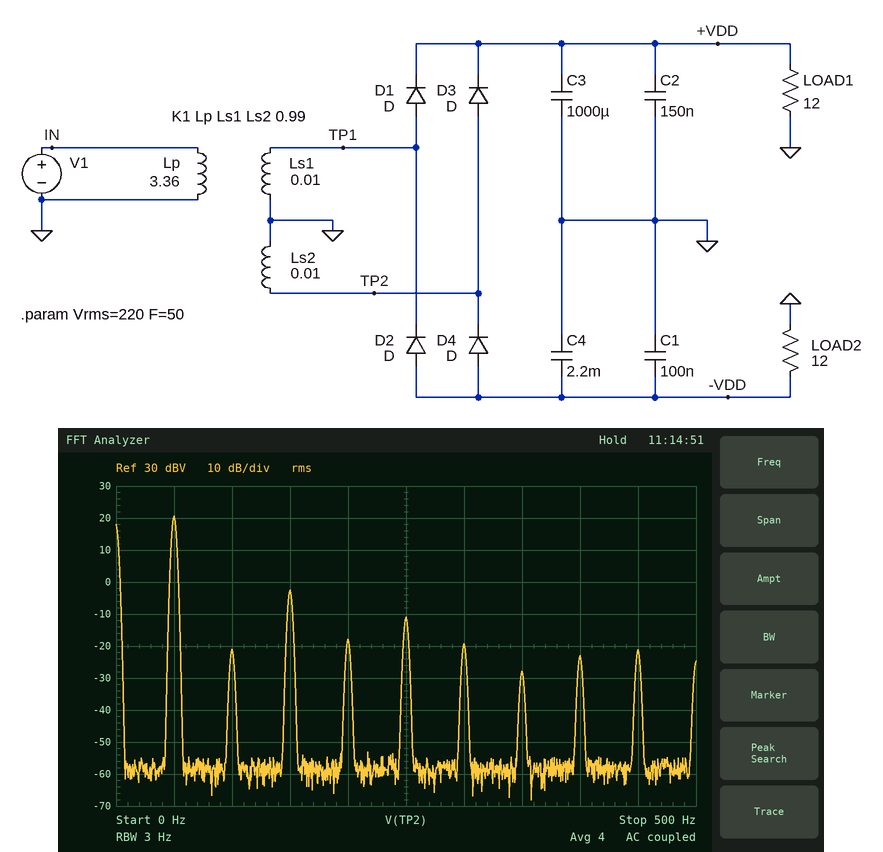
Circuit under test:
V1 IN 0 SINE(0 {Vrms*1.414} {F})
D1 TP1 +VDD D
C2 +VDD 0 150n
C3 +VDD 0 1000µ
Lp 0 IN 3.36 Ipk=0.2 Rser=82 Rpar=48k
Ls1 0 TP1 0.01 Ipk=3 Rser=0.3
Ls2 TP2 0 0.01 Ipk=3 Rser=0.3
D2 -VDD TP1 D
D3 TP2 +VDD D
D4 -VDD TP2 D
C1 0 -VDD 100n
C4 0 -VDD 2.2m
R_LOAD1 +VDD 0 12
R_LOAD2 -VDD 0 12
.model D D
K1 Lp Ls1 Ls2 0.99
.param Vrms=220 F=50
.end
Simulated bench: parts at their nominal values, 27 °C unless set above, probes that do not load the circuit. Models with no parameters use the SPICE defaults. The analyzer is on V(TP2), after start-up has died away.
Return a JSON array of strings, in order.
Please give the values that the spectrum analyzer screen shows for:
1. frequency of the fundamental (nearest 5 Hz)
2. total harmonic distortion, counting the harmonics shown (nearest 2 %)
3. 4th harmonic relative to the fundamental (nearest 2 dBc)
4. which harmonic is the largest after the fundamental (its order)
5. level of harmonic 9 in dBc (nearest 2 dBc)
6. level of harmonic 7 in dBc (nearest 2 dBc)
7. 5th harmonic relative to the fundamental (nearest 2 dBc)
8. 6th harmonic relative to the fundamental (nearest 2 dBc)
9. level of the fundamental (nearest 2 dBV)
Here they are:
["50 Hz", "8 %", "-38 dBc", "3", "-42 dBc", "-48 dBc", "-32 dBc", "-40 dBc", "20 dBV"]
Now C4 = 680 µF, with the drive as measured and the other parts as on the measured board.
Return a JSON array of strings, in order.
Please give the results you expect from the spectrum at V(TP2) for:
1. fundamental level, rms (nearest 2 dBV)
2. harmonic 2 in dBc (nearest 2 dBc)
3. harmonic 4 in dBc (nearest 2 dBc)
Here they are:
["20 dBV", "-50 dBc", "-46 dBc"]
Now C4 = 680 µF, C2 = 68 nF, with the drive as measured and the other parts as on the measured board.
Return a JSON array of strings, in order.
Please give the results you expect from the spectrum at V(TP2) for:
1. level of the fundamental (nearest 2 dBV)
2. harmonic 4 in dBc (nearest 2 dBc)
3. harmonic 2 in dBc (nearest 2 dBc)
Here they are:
["20 dBV", "-46 dBc", "-50 dBc"]
